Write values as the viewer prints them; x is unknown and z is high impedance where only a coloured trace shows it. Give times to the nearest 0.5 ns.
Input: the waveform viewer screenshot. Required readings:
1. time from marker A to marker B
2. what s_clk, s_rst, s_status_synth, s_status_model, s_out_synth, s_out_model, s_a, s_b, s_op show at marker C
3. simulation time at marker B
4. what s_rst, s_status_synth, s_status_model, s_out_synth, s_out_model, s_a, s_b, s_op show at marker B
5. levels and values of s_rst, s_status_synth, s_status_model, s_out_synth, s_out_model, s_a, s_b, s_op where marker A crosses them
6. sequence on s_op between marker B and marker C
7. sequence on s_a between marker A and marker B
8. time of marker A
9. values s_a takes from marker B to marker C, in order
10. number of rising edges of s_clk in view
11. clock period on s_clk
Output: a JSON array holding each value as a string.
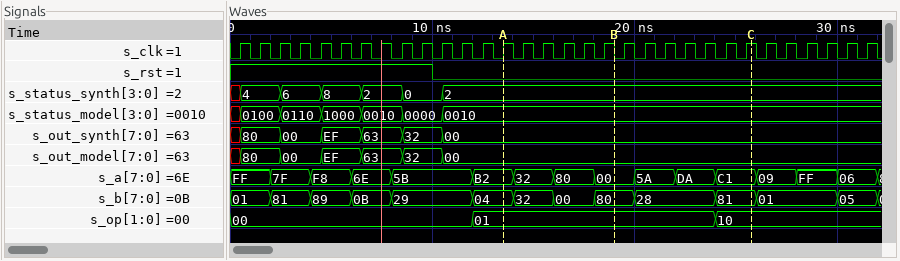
["5.5 ns", "s_clk=1, s_rst=0, s_status_synth=2, s_status_model=0010, s_out_synth=00, s_out_model=00, s_a=C1, s_b=81, s_op=10", "19 ns", "s_rst=0, s_status_synth=2, s_status_model=0010, s_out_synth=00, s_out_model=00, s_a=00, s_b=80, s_op=01", "s_rst=0, s_status_synth=2, s_status_model=0010, s_out_synth=00, s_out_model=00, s_a=B2, s_b=04, s_op=01", "01, 10", "B2, 32, 80, 00", "13.5 ns", "00, 5A, DA, C1", "32", "1 ns"]
